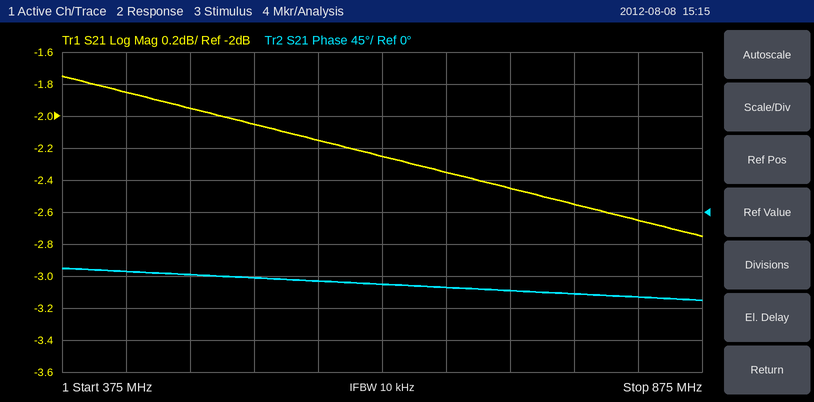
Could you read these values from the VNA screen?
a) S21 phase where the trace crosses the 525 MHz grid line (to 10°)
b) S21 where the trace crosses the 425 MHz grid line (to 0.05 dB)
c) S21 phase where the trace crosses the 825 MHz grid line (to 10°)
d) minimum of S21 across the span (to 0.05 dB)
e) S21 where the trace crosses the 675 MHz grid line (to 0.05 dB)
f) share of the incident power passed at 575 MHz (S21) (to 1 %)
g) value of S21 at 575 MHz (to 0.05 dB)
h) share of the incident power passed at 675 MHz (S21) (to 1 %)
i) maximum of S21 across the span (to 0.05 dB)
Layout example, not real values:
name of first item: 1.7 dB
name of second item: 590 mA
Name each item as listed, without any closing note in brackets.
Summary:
S21 phase where the trace crosses the 525 MHz grid line: -90°
S21 where the trace crosses the 425 MHz grid line: -1.85 dB
S21 phase where the trace crosses the 825 MHz grid line: -120°
minimum of S21 across the span: -2.75 dB
S21 where the trace crosses the 675 MHz grid line: -2.35 dB
share of the incident power passed at 575 MHz (S21): 61 %
value of S21 at 575 MHz: -2.15 dB
share of the incident power passed at 675 MHz (S21): 58 %
maximum of S21 across the span: -1.75 dB
